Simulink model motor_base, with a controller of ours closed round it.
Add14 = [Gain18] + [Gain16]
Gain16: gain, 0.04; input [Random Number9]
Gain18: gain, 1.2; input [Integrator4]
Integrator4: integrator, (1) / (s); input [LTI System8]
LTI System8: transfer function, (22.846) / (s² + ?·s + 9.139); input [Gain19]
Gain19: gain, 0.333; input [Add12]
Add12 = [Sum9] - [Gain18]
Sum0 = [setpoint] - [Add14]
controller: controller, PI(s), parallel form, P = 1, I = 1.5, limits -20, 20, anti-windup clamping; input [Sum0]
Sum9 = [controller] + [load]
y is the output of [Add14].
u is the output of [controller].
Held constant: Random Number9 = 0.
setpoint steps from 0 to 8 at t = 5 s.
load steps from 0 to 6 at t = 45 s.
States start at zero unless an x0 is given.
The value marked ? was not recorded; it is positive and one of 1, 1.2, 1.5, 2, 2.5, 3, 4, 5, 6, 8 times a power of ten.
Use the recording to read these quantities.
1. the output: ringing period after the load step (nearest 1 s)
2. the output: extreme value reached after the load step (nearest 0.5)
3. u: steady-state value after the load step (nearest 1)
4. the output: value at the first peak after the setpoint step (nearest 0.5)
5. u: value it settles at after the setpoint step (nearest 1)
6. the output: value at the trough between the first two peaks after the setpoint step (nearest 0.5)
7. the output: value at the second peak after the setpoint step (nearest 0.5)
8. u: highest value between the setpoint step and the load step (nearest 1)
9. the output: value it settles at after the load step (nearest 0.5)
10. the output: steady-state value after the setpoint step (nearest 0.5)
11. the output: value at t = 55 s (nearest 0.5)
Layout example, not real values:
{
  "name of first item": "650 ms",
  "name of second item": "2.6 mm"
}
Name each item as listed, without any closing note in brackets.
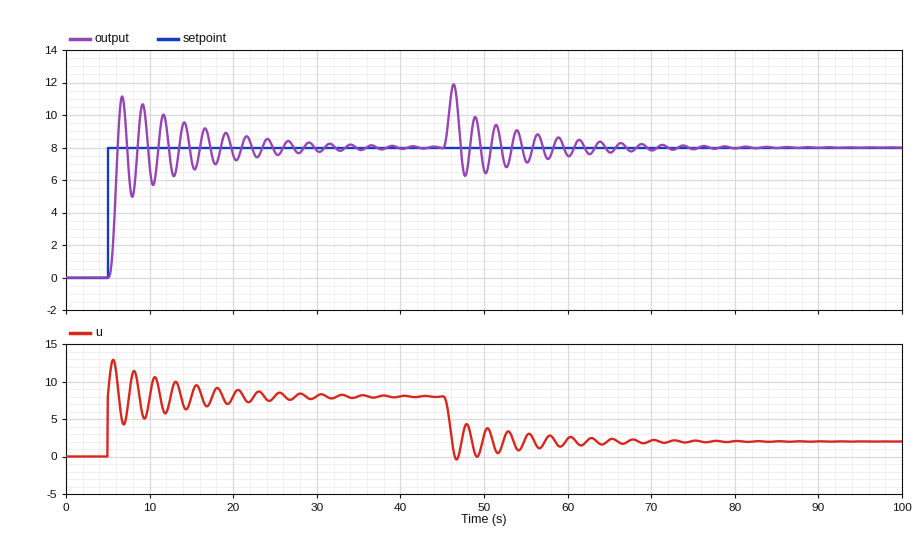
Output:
{
  "the output: ringing period after the load step": "3 s",
  "the output: extreme value reached after the load step": "12.0",
  "u: steady-state value after the load step": "2",
  "the output: value at the first peak after the setpoint step": "11.0",
  "u: value it settles at after the setpoint step": "8",
  "the output: value at the trough between the first two peaks after the setpoint step": "5.0",
  "the output: value at the second peak after the setpoint step": "10.5",
  "u: highest value between the setpoint step and the load step": "13",
  "the output: value it settles at after the load step": "8.0",
  "the output: steady-state value after the setpoint step": "8.0",
  "the output: value at t = 55 s": "7.0"
}
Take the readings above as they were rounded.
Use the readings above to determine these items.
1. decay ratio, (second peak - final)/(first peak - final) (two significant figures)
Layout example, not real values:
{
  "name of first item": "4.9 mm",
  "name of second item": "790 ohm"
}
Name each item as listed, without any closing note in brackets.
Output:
{
  "decay ratio, (second peak - final)/(first peak - final)": "0.83"
}
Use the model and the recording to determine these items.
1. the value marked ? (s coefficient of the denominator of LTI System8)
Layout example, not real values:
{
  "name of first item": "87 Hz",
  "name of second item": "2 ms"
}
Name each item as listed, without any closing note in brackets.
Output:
{
  "the value marked ?": "3"
}
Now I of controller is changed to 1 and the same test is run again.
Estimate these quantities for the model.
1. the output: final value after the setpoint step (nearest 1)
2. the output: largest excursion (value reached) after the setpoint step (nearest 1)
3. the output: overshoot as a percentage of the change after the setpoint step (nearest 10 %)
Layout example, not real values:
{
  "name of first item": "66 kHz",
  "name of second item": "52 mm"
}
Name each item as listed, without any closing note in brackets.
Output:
{
  "the output: final value after the setpoint step": "8",
  "the output: largest excursion (value reached) after the setpoint step": "9",
  "the output: overshoot as a percentage of the change after the setpoint step": "20 %"
}
